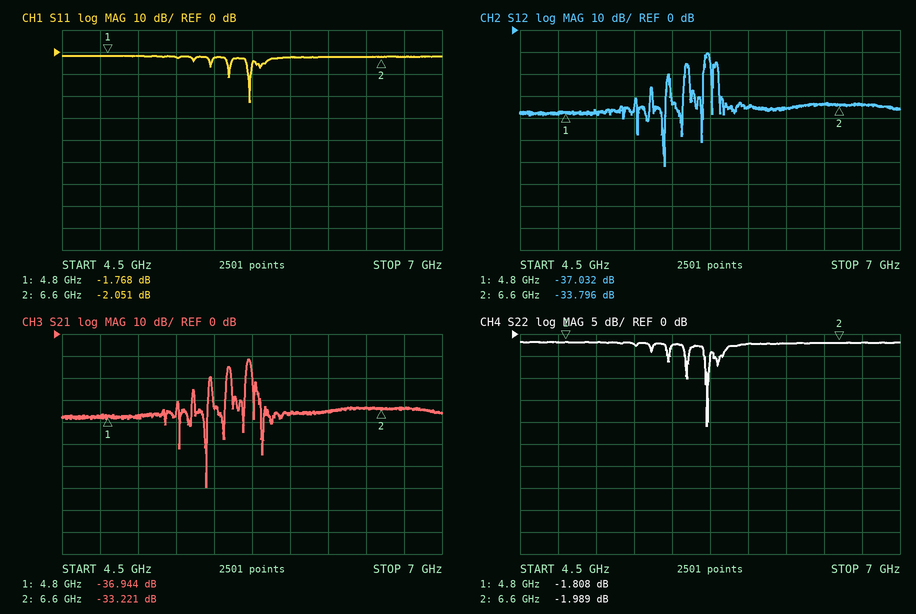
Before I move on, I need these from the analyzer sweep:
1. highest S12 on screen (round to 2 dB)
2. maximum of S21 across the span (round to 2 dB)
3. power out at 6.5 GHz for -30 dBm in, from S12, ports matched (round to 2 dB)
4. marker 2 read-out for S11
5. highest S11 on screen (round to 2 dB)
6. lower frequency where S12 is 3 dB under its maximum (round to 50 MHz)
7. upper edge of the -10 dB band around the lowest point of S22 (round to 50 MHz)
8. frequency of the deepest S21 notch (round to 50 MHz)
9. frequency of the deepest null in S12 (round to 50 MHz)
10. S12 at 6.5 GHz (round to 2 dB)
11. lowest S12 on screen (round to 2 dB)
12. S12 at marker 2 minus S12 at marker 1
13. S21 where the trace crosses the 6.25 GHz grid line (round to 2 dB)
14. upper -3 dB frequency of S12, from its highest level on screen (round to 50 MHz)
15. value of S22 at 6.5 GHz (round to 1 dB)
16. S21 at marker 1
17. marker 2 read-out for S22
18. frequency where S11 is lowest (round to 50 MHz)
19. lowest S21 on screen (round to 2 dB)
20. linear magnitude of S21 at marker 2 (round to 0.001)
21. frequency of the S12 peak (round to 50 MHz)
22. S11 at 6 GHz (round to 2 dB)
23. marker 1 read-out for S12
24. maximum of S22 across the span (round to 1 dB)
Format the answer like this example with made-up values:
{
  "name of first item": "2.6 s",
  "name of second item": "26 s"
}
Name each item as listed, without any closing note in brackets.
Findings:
{
  "highest S12 on screen": "-10 dB",
  "maximum of S21 across the span": "-12 dB",
  "power out at 6.5 GHz for -30 dBm in, from S12, ports matched": "-64 dBm",
  "marker 2 read-out for S11": "-2.051 dB",
  "highest S11 on screen": "-2 dB",
  "lower frequency where S12 is 3 dB under its maximum": "5.70 GHz",
  "upper edge of the -10 dB band around the lowest point of S22": "5.75 GHz",
  "frequency of the deepest S21 notch": "5.45 GHz",
  "frequency of the deepest null in S12": "5.45 GHz",
  "S12 at 6.5 GHz": "-34 dB",
  "lowest S12 on screen": "-62 dB",
  "S12 at marker 2 minus S12 at marker 1": "3.236 dB",
  "S21 where the trace crosses the 6.25 GHz grid line": "-36 dB",
  "upper -3 dB frequency of S12, from its highest level on screen": "5.75 GHz",
  "value of S22 at 6.5 GHz": "-2 dB",
  "S21 at marker 1": "-36.944 dB",
  "marker 2 read-out for S22": "-1.989 dB",
  "frequency where S11 is lowest": "5.75 GHz",
  "lowest S21 on screen": "-70 dB",
  "linear magnitude of S21 at marker 2": "0.022",
  "frequency of the S12 peak": "5.75 GHz",
  "S11 at 6 GHz": "-2 dB",
  "marker 1 read-out for S12": "-37.032 dB",
  "maximum of S22 across the span": "-2 dB"
}
